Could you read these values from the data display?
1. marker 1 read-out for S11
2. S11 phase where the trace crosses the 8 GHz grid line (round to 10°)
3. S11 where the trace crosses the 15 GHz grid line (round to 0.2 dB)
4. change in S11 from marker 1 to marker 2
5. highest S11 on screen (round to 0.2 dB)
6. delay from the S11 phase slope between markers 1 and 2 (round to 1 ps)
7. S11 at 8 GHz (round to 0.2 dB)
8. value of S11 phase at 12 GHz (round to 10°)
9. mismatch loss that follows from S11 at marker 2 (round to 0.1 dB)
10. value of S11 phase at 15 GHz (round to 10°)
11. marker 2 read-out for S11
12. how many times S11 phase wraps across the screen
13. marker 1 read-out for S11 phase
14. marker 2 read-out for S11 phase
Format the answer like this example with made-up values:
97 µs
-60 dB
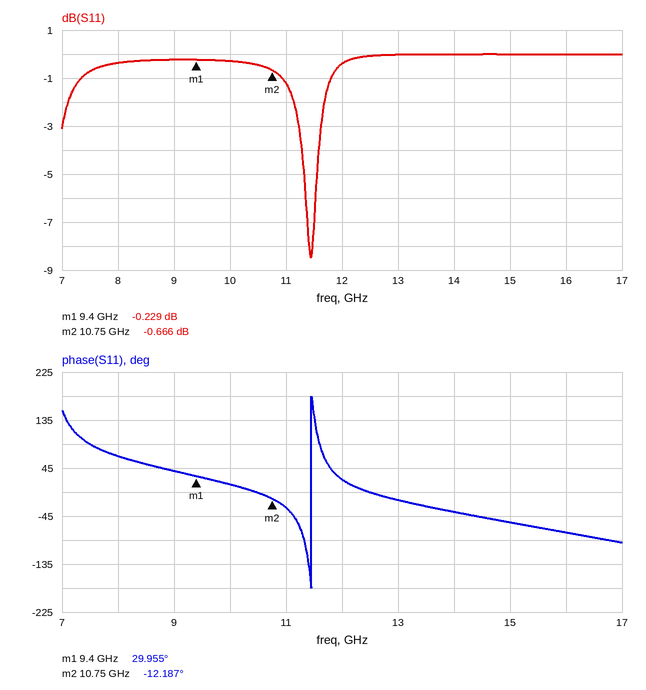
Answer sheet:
-0.229 dB
70°
0.0 dB
-0.437 dB
0.0 dB
87 ps
-0.4 dB
20°
8.5 dB
-60°
-0.666 dB
1
29.955°
-12.187°
